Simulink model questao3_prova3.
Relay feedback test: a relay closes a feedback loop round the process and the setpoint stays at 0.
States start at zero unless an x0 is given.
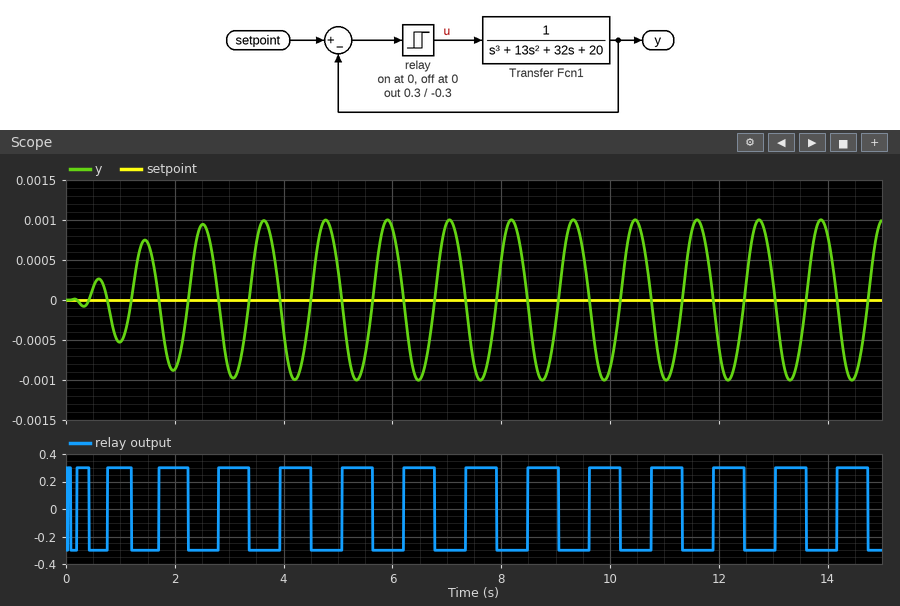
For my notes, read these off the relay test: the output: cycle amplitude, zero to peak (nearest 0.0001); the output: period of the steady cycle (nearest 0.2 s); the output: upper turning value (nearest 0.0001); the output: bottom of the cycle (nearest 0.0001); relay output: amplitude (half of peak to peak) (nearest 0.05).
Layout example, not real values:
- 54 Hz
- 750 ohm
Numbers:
- 0.0010
- 1.2 s
- 0.0010
- -0.0010
- 0.30
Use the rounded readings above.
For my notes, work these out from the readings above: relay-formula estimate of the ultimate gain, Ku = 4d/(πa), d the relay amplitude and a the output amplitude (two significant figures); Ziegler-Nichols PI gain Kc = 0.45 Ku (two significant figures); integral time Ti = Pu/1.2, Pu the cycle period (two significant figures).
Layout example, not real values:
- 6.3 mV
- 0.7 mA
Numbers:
- 380
- 170
- 1.0 s
